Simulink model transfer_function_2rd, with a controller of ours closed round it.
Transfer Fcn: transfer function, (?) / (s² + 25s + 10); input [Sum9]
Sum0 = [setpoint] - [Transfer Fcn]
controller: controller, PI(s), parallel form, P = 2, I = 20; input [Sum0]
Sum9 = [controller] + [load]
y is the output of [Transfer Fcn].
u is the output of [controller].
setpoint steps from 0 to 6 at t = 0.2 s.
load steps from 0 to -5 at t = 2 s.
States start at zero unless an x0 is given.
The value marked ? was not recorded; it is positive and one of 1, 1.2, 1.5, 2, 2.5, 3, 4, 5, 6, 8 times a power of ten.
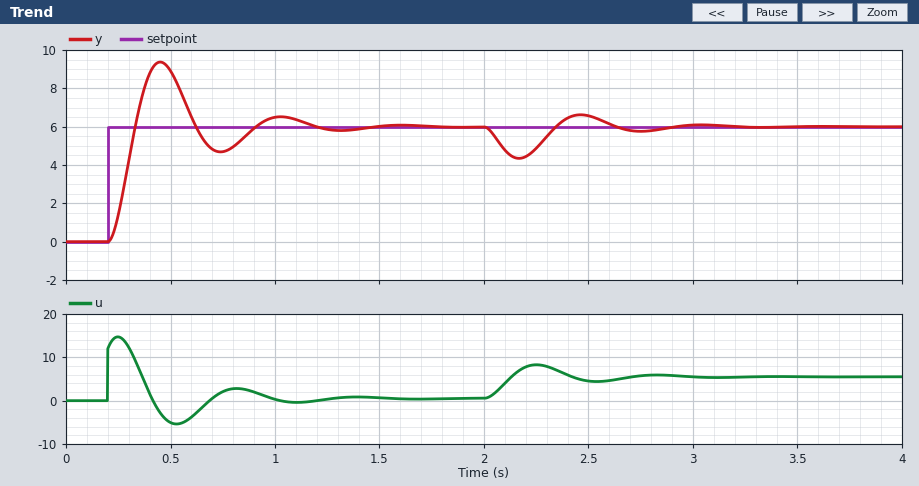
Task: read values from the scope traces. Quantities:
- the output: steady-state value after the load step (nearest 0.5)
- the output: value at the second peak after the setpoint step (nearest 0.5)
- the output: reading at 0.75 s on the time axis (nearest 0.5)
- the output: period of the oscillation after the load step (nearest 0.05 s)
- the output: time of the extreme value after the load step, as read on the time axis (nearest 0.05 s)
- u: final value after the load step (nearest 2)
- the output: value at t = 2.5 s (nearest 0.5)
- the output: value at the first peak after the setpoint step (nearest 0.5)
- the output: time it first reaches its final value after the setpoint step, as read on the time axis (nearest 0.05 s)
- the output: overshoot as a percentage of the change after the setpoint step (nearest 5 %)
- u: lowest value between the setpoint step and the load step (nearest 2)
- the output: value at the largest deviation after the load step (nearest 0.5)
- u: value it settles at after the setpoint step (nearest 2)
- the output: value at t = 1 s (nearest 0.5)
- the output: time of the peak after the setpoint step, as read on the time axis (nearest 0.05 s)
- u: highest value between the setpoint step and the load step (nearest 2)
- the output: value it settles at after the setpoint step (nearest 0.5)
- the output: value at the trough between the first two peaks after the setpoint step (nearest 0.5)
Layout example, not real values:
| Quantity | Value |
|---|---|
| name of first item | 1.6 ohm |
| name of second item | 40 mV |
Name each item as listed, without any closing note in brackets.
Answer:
| Quantity | Value |
|---|---|
| the output: steady-state value after the load step | 6.0 |
| the output: value at the second peak after the setpoint step | 6.5 |
| the output: reading at 0.75 s on the time axis | 4.5 |
| the output: period of the oscillation after the load step | 0.60 s |
| the output: time of the extreme value after the load step, as read on the time axis | 2.15 s |
| u: final value after the load step | 6 |
| the output: value at t = 2.5 s | 6.5 |
| the output: value at the first peak after the setpoint step | 9.5 |
| the output: time it first reaches its final value after the setpoint step, as read on the time axis | 0.35 s |
| the output: overshoot as a percentage of the change after the setpoint step | 55 % |
| u: lowest value between the setpoint step and the load step | -6 |
| the output: value at the largest deviation after the load step | 4.5 |
| u: value it settles at after the setpoint step | 0 |
| the output: value at t = 1 s | 6.5 |
| the output: time of the peak after the setpoint step, as read on the time axis | 0.45 s |
| u: highest value between the setpoint step and the load step | 14 |
| the output: value it settles at after the setpoint step | 6.0 |
| the output: value at the trough between the first two peaks after the setpoint step | 4.5 |
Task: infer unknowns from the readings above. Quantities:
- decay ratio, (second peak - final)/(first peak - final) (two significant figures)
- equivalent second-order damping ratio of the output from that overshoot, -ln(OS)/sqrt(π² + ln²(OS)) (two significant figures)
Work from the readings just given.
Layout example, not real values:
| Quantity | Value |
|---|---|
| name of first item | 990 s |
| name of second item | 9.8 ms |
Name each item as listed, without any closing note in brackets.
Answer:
| Quantity | Value |
|---|---|
| decay ratio, (second peak - final)/(first peak - final) | 0.14 |
| equivalent second-order damping ratio of the output from that overshoot, -ln(OS)/sqrt(π² + ln²(OS)) | 0.19 |
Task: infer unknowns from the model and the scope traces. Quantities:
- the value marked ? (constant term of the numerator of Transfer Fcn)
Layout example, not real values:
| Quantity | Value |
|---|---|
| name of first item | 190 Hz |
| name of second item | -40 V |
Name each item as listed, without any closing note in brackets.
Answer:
| Quantity | Value |
|---|---|
| the value marked ? | 120 |
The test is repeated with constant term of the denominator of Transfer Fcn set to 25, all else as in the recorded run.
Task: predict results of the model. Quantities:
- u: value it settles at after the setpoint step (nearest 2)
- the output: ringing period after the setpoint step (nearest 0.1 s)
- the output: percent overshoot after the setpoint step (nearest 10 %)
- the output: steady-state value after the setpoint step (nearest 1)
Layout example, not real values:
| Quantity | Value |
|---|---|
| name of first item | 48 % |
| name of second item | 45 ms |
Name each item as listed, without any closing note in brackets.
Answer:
| Quantity | Value |
|---|---|
| u: value it settles at after the setpoint step | 2 |
| the output: ringing period after the setpoint step | 0.6 s |
| the output: percent overshoot after the setpoint step | 50 % |
| the output: steady-state value after the setpoint step | 6 |
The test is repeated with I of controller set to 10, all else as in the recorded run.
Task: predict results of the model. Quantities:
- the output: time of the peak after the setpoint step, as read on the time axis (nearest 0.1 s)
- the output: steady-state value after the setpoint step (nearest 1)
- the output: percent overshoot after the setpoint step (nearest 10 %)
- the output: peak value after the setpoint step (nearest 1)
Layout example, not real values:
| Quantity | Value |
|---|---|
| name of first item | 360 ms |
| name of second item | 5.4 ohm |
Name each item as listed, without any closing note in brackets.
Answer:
| Quantity | Value |
|---|---|
| the output: time of the peak after the setpoint step, as read on the time axis | 0.5 s |
| the output: steady-state value after the setpoint step | 6 |
| the output: percent overshoot after the setpoint step | 30 % |
| the output: peak value after the setpoint step | 8 |
